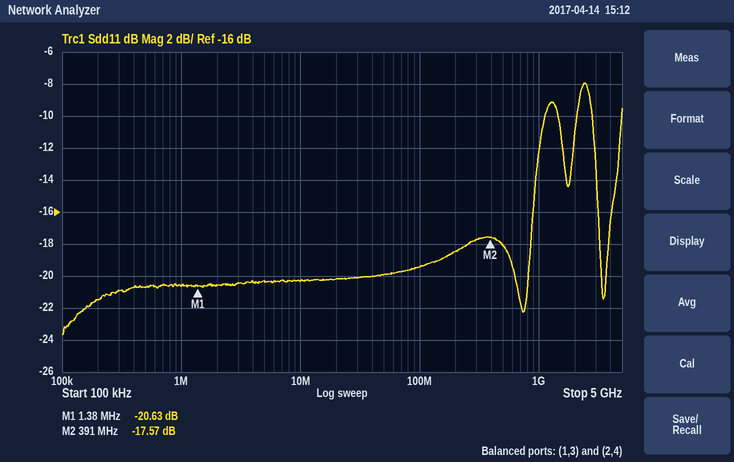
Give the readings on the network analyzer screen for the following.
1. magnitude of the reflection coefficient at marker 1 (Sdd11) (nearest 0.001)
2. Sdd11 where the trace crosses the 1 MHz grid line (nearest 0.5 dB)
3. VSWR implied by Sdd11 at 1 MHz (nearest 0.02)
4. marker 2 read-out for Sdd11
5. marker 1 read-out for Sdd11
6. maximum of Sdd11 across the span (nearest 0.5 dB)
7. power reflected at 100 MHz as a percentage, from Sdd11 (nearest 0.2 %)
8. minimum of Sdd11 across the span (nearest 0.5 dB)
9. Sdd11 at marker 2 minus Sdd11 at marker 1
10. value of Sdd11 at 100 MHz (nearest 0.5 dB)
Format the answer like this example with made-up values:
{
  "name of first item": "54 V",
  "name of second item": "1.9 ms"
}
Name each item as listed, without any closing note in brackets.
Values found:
{
  "magnitude of the reflection coefficient at marker 1 (Sdd11)": "0.093",
  "Sdd11 where the trace crosses the 1 MHz grid line": "-20.5 dB",
  "VSWR implied by Sdd11 at 1 MHz": "1.20",
  "marker 2 read-out for Sdd11": "-17.57 dB",
  "marker 1 read-out for Sdd11": "-20.63 dB",
  "maximum of Sdd11 across the span": "-8.0 dB",
  "power reflected at 100 MHz as a percentage, from Sdd11": "1.2 %",
  "minimum of Sdd11 across the span": "-23.5 dB",
  "Sdd11 at marker 2 minus Sdd11 at marker 1": "3.06 dB",
  "value of Sdd11 at 100 MHz": "-19.5 dB"
}
